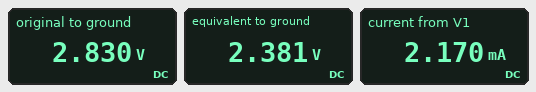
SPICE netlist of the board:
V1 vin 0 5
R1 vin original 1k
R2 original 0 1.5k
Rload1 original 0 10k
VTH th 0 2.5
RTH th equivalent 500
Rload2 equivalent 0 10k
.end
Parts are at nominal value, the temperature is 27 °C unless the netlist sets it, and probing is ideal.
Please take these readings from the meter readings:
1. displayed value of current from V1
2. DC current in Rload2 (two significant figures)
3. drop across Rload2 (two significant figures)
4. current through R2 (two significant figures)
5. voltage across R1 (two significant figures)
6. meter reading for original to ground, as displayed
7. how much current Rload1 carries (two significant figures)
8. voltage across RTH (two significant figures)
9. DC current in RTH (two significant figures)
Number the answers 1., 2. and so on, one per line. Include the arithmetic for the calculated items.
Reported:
1. 2.170 mA
2. (2.381 V) / 10 kΩ = 240 µA
3. 2.381 V = 2.4 V
4. (2.83 V) / 1.5 kΩ = 1.9 mA
5. 5 V - 2.83 V = 2.2 V
6. 2.830 V
7. (2.83 V) / 10 kΩ = 280 µA
8. 2.5 V - 2.381 V = 120 mV
9. (2.5 V - 2.381 V) / 500 Ω = 240 µA
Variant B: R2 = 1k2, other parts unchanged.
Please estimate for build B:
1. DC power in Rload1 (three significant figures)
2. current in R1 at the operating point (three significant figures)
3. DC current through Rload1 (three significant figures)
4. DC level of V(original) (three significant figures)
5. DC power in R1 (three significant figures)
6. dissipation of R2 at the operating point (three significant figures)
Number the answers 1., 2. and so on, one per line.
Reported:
1. 669 µW
2. 2.41 mA
3. 259 µA
4. 2.59 V
5. 5.83 mW
6. 5.57 mW
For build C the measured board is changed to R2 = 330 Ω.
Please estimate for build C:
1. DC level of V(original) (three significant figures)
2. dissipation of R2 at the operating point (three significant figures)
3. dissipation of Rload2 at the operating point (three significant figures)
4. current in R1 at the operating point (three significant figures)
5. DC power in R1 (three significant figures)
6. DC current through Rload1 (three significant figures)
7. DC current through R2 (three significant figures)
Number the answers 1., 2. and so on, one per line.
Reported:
1. 1.21 V
2. 4.44 mW
3. 567 µW
4. 3.79 mA
5. 14.4 mW
6. 121 µA
7. 3.67 mA
